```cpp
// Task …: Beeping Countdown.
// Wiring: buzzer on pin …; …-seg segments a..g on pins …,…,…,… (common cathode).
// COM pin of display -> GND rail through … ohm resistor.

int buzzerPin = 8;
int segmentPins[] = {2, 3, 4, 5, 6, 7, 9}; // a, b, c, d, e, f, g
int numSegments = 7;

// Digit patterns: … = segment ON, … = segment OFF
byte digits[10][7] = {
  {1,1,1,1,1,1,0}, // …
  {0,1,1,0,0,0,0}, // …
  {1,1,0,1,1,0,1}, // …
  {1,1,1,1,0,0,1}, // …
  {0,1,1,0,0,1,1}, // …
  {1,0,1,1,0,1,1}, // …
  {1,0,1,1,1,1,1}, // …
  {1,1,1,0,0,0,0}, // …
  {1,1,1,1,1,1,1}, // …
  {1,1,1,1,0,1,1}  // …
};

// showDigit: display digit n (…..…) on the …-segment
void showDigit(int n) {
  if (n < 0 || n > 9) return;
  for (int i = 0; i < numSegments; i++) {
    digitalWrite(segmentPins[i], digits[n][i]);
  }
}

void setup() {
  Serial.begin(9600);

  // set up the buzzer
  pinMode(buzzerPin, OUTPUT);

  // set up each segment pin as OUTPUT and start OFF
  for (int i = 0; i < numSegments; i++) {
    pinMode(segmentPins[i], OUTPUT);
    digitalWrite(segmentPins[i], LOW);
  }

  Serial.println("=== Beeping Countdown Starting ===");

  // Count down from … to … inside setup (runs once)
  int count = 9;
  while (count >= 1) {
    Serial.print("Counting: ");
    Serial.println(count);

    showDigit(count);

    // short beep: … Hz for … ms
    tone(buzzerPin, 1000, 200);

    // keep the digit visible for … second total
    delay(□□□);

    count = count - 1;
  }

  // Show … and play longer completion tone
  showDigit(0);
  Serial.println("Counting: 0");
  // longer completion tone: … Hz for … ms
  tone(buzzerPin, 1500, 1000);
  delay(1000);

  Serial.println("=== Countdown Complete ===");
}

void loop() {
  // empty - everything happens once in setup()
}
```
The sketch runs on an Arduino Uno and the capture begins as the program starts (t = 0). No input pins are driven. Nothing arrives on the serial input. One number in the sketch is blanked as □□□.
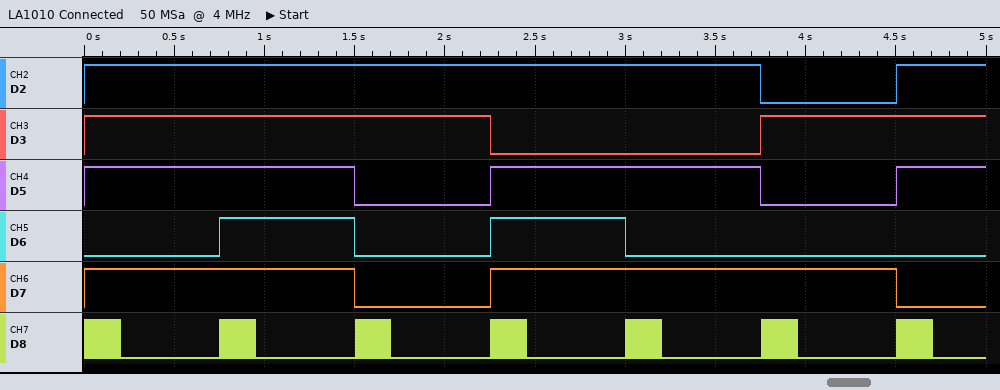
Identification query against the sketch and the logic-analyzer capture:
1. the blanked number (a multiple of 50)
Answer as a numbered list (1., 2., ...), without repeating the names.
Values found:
1. 750
